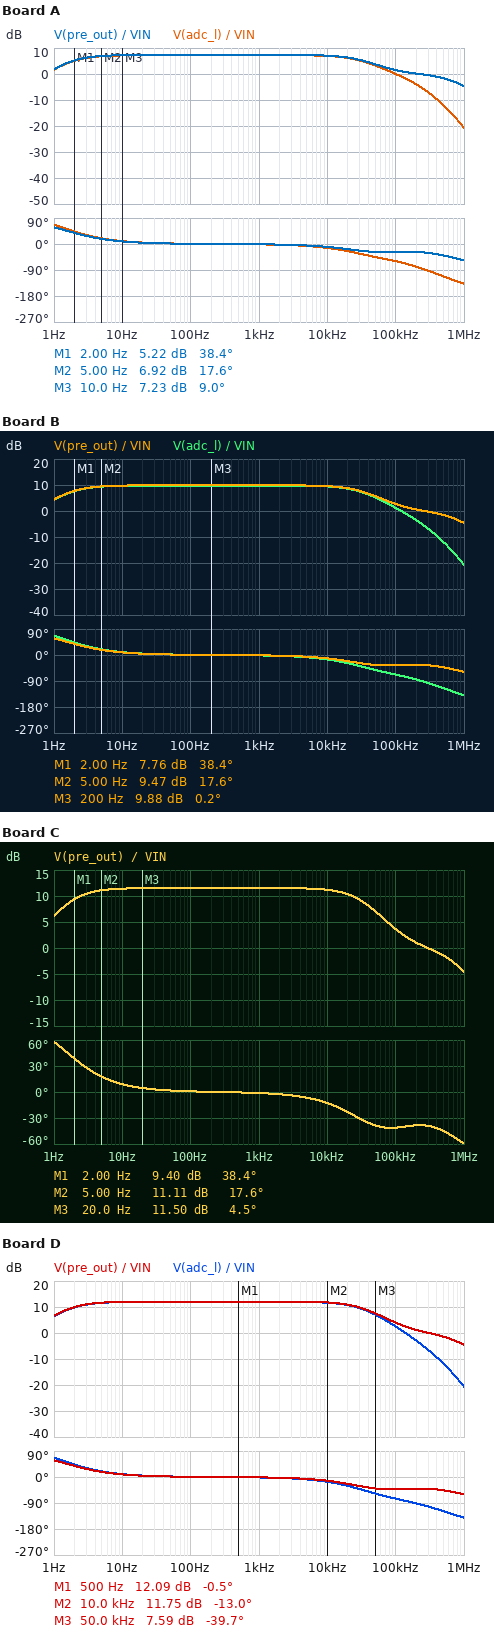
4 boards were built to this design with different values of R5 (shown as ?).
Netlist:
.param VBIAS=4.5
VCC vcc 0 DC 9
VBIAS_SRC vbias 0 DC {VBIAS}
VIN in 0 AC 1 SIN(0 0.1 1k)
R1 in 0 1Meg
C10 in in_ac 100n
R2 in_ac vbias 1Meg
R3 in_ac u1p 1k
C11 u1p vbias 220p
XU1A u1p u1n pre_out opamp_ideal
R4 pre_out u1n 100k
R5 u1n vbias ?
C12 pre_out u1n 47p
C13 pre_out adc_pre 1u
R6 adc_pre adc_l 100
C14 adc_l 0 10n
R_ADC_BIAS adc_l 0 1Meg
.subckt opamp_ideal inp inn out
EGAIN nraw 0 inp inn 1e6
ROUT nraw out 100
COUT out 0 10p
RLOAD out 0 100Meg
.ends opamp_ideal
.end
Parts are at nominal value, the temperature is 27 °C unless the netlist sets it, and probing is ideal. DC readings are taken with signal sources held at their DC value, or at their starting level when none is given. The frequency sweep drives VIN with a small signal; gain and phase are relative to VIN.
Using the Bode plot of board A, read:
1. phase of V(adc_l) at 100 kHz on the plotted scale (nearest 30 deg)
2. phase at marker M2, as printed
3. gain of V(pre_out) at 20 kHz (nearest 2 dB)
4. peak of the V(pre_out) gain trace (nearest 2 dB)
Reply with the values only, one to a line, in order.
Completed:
-60 deg
17.6 deg
6 dB
8 dB
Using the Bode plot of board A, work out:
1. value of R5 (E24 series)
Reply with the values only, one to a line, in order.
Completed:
75 kΩ
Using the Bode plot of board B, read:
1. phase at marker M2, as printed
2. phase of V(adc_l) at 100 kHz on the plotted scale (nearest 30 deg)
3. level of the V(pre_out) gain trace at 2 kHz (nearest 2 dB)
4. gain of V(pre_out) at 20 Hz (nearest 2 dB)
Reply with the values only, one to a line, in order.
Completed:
17.6 deg
-60 deg
10 dB
10 dB
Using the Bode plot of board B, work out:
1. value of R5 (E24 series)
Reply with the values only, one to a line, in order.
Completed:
47 kΩ
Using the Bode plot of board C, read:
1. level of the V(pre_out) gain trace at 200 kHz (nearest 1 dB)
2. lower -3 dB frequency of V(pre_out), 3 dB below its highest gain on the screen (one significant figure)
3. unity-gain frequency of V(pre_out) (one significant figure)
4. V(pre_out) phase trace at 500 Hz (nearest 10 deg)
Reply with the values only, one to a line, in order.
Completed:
1 dB
2 Hz
300 kHz
0 deg
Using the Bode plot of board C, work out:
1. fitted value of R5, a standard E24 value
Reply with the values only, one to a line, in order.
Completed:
36 kΩ
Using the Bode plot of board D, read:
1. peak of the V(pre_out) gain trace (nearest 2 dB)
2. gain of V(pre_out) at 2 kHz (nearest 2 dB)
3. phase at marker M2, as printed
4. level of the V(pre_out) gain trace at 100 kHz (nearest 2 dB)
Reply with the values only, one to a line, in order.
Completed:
12 dB
12 dB
-13.0 deg
4 dB
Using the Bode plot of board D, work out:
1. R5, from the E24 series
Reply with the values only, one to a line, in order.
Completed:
33 kΩ
